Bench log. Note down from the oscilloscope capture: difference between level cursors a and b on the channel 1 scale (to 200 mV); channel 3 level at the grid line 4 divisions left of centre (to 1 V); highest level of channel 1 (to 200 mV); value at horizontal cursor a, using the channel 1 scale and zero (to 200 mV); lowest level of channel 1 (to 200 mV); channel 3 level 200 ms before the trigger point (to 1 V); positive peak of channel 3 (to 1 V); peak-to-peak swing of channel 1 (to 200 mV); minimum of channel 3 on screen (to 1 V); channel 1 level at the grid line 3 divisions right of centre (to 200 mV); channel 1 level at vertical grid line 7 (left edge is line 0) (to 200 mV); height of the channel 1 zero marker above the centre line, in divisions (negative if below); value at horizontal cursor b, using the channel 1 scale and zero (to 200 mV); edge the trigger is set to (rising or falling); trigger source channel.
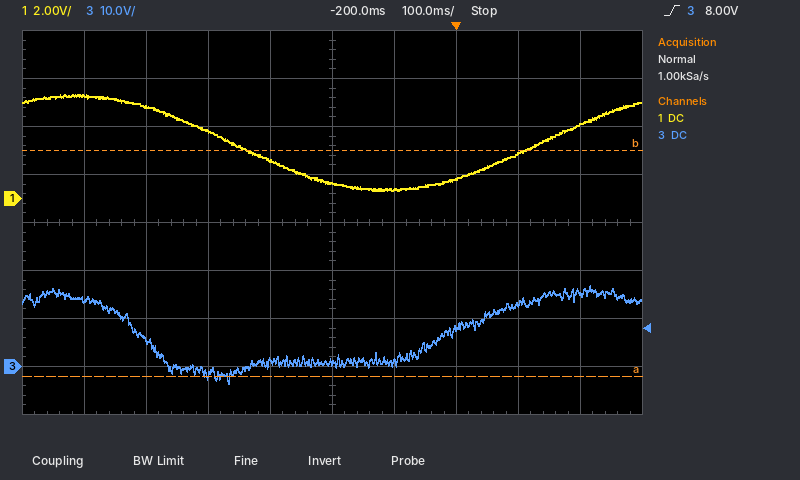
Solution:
9.4 V
14 V
4.4 V
-7.4 V
400 mV
1 V
17 V
4.0 V
-4 V
1.8 V
800 mV
+0.5 div
2.0 V
rising
channel 3
